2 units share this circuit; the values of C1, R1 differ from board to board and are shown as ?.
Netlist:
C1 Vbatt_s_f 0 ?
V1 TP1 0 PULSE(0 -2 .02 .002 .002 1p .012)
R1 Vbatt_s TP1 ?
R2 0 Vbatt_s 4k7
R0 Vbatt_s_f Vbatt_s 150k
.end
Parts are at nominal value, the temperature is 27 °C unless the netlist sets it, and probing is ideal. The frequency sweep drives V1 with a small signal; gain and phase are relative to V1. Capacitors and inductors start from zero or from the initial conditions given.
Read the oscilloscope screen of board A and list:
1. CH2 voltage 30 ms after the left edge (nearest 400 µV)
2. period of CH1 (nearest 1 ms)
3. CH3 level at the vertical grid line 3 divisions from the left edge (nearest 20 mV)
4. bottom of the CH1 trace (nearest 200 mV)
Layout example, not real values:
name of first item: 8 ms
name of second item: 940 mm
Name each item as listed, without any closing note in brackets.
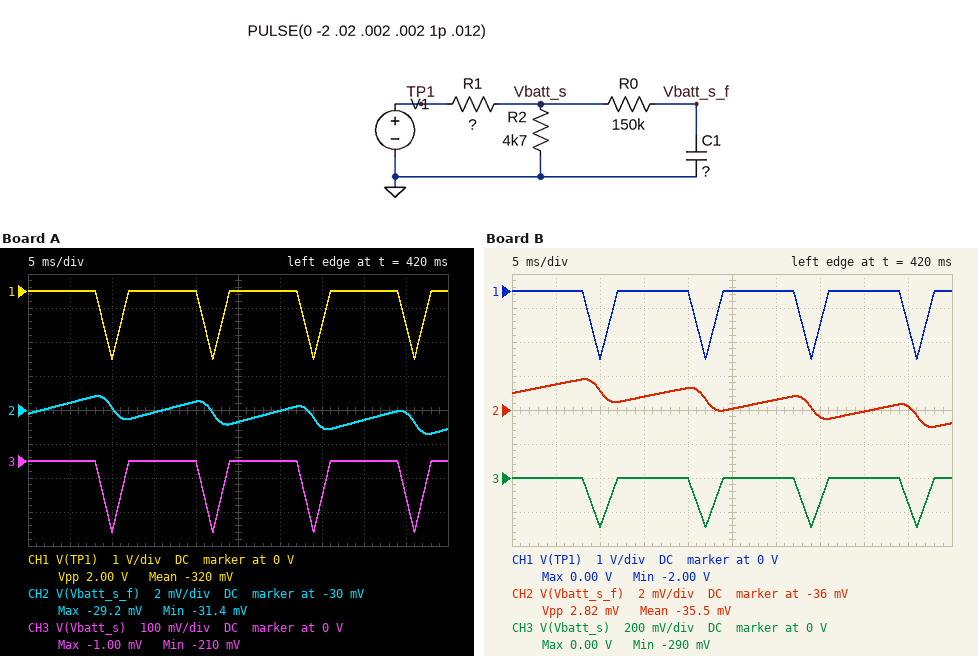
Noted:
CH2 voltage 30 ms after the left edge: -30.0 mV
period of CH1: 12 ms
CH3 level at the vertical grid line 3 divisions from the left edge: 0 V
bottom of the CH1 trace: -2.0 V
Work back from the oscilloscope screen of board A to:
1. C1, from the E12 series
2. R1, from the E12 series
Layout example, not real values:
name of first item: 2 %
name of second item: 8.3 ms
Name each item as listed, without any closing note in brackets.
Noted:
C1, from the E12 series: 1.5 µF
R1, from the E12 series: 39 kΩ
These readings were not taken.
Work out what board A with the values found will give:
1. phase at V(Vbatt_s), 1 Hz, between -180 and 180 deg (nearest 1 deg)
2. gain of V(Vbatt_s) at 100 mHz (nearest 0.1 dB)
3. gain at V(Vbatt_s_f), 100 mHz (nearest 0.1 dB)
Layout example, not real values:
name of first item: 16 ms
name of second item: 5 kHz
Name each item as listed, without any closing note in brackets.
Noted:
phase at V(Vbatt_s), 1 Hz, between -180 and 180 deg: -1 deg
gain of V(Vbatt_s) at 100 mHz: -19.4 dB
gain at V(Vbatt_s_f), 100 mHz: -19.5 dB
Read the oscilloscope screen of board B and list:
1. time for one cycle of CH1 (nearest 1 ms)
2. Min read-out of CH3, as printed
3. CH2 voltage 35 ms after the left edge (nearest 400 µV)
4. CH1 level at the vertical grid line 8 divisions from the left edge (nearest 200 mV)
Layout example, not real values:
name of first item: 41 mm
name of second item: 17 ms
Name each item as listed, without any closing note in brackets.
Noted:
time for one cycle of CH1: 12 ms
Min read-out of CH3, as printed: -290 mV
CH2 voltage 35 ms after the left edge: -36.4 mV
CH1 level at the vertical grid line 8 divisions from the left edge: 0 V
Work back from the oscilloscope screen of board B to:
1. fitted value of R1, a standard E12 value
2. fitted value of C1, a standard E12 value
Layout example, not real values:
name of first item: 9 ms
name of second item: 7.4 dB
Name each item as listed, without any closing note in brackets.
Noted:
fitted value of R1, a standard E12 value: 27 kΩ
fitted value of C1, a standard E12 value: 2.2 µF
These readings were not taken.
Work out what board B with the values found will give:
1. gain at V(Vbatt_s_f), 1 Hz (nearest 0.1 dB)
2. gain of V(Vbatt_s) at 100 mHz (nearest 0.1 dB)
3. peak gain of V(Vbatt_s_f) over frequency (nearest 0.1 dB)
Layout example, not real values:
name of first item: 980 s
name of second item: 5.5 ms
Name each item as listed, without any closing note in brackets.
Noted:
gain at V(Vbatt_s_f), 1 Hz: -24.0 dB
gain of V(Vbatt_s) at 100 mHz: -16.6 dB
peak gain of V(Vbatt_s_f) over frequency: -16.6 dB
